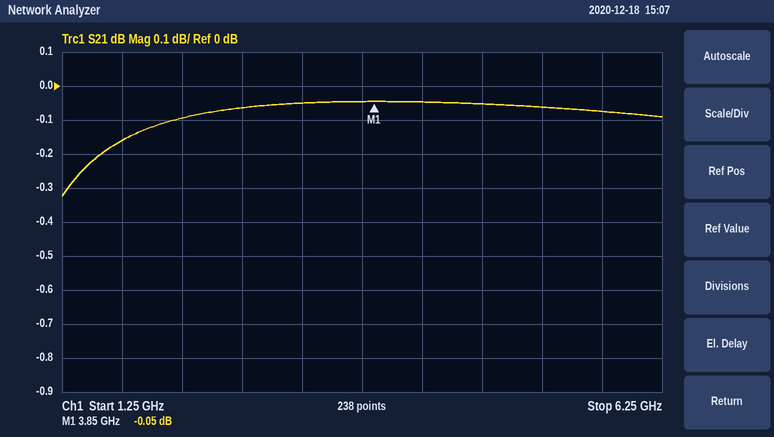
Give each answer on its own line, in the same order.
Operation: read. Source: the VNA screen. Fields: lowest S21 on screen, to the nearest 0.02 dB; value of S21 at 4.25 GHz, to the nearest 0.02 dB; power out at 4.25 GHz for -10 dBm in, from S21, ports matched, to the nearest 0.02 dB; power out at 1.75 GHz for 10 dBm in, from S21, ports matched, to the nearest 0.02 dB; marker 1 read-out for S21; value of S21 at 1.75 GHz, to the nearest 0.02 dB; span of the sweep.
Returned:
-0.32 dB
-0.04 dB
-10.04 dBm
9.84 dBm
-0.05 dB
-0.16 dB
5 GHz
